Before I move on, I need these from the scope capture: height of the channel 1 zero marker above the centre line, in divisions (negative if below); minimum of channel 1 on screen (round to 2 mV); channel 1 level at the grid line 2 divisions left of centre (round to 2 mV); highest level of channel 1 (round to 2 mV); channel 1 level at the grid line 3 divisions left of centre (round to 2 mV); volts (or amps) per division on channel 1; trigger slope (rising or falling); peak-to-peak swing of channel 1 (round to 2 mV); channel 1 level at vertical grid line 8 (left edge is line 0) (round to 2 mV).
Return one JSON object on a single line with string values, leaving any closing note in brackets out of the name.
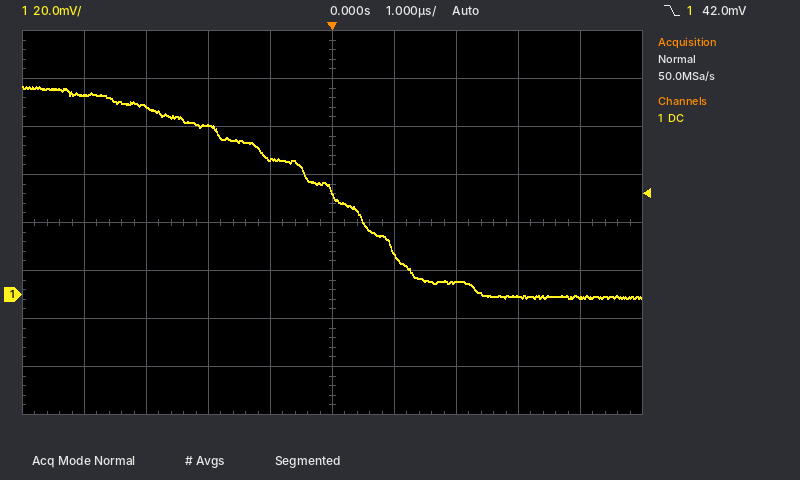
{"height of the channel 1 zero marker above the centre line, in divisions": "-1.5 div", "minimum of channel 1 on screen": "-2 mV", "channel 1 level at the grid line 2 divisions left of centre": "70 mV", "highest level of channel 1": "86 mV", "channel 1 level at the grid line 3 divisions left of centre": "78 mV", "volts (or amps) per division on channel 1": "20 mV", "trigger slope": "falling", "peak-to-peak swing of channel 1": "88 mV", "channel 1 level at vertical grid line 8 (left edge is line 0)": "0 mV"}
